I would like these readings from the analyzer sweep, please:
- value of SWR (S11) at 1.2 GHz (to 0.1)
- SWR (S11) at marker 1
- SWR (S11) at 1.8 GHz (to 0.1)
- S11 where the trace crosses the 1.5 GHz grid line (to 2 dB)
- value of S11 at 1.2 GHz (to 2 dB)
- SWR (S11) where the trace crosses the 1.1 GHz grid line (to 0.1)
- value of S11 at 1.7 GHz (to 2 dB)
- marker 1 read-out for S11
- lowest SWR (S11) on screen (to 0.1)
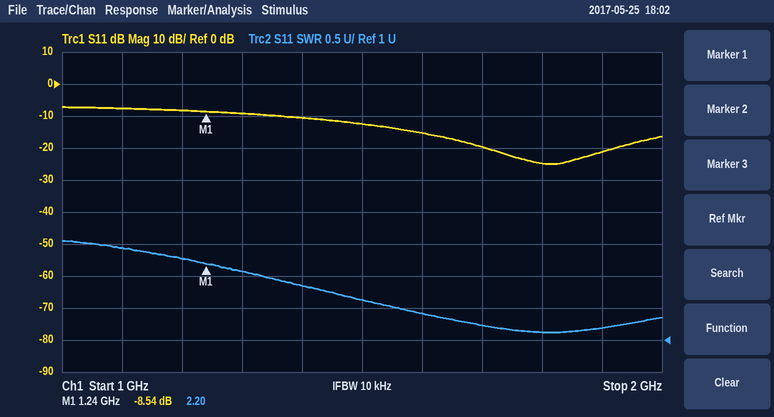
2.3
2.20
1.1
-12 dB
-8 dB
2.4
-20 dB
-8.54 dB
1.1
